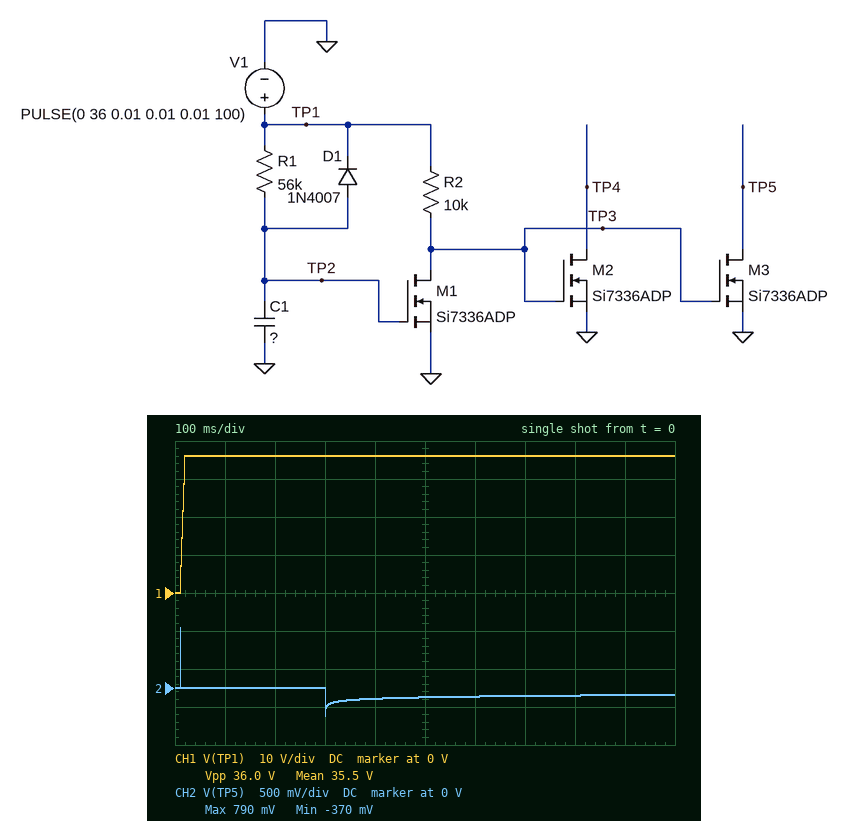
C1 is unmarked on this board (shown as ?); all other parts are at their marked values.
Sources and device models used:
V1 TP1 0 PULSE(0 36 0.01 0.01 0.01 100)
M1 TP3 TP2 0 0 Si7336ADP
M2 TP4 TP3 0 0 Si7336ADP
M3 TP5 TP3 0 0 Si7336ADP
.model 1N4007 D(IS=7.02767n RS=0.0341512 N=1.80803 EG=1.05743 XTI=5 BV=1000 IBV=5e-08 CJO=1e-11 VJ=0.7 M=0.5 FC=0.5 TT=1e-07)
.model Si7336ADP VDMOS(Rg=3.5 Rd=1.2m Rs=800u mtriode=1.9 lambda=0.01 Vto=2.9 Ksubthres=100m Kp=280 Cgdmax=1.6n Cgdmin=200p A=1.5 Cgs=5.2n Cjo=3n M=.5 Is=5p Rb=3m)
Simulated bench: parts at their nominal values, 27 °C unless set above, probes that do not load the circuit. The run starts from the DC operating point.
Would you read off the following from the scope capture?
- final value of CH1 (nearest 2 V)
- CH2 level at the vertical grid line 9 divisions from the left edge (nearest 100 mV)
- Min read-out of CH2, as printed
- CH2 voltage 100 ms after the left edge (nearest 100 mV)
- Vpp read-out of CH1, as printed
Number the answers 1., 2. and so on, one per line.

1. 36 V
2. -100 mV
3. -370 mV
4. 0 V
5. 36.0 V
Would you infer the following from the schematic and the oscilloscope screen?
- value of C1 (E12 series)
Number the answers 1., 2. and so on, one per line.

1. 68 µF
